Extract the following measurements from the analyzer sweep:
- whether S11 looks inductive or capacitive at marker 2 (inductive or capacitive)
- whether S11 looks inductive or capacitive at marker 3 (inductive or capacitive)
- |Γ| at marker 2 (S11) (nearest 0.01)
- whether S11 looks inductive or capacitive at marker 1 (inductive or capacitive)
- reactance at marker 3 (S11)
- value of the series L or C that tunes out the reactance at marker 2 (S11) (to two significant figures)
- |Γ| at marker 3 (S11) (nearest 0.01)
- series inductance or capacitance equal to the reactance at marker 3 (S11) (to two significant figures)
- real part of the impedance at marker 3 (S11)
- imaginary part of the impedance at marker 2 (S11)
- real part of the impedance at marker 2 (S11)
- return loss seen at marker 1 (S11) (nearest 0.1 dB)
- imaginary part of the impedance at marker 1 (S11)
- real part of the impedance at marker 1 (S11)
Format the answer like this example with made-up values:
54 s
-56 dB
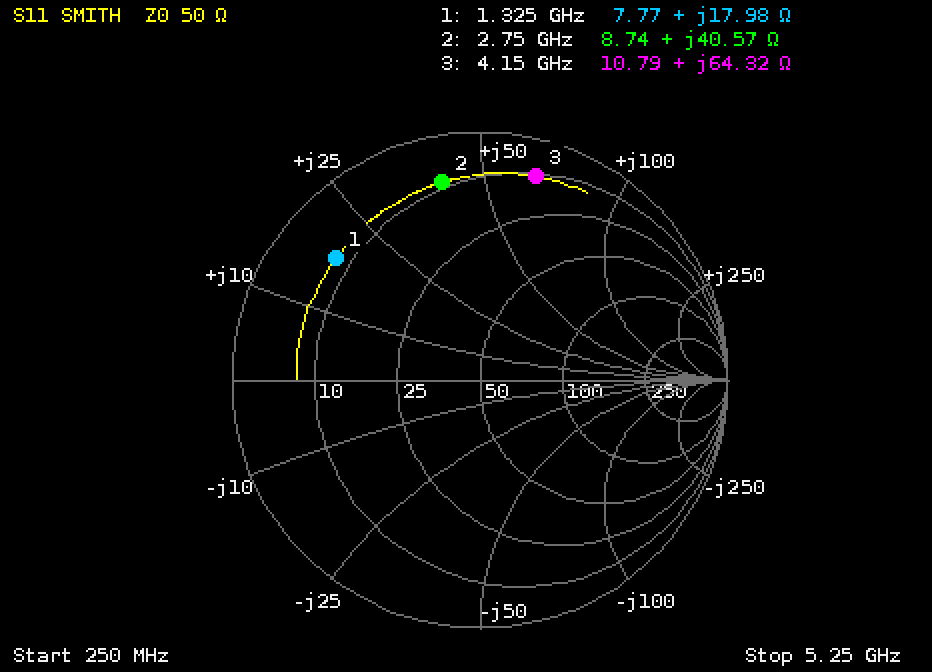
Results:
inductive
inductive
0.81
inductive
+64.32 Ω
1.4 pF
0.85
2.5 nH
10.79 Ω
+40.57 Ω
8.74 Ω
2.4 dB
+17.98 Ω
7.77 Ω
